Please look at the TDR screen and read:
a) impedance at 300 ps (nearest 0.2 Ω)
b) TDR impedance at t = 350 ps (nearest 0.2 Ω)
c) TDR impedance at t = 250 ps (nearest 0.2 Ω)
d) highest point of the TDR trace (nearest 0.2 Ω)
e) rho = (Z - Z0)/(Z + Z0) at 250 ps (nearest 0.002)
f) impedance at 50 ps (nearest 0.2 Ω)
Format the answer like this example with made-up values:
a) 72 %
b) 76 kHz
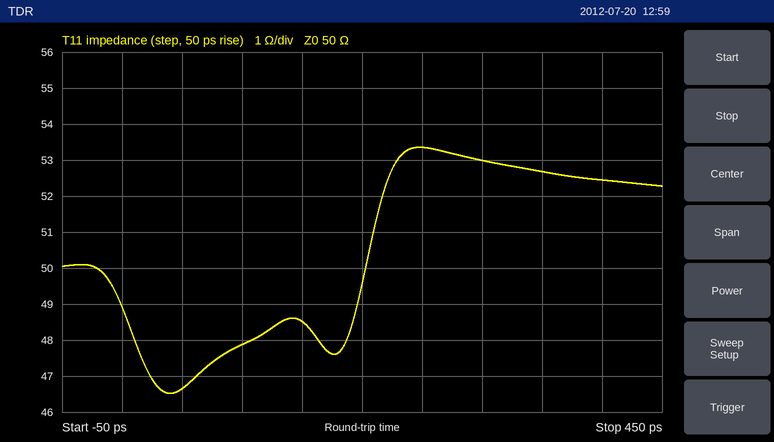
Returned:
a) 53.0 Ω
b) 52.6 Ω
c) 53.4 Ω
d) 53.4 Ω
e) +0.032
f) 46.6 Ω
